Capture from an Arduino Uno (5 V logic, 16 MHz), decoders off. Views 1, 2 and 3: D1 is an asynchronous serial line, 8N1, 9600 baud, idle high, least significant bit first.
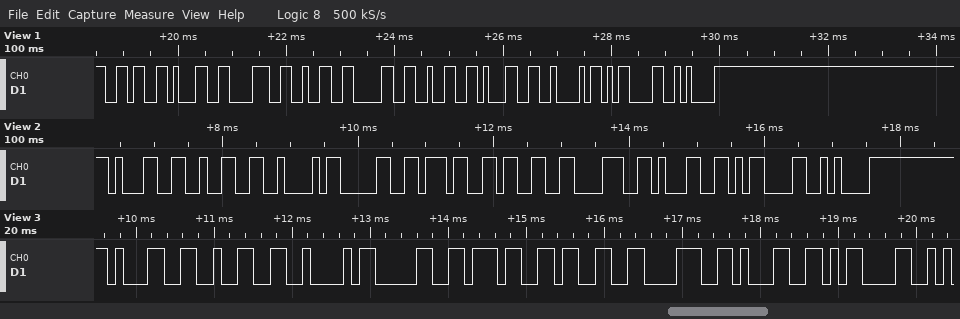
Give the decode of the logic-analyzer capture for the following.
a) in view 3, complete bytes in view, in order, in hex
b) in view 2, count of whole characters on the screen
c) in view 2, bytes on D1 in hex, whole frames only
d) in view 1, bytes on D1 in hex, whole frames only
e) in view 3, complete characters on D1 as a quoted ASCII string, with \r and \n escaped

0x31 0x32 0x42 0x30 0x37 0x33 0x38 0x31 0x0D
10
31 32 42 30 37 33 38 31 0D 0A
36 31 38 32 30 32 31 42 0D 0A
"12B07381\r"
